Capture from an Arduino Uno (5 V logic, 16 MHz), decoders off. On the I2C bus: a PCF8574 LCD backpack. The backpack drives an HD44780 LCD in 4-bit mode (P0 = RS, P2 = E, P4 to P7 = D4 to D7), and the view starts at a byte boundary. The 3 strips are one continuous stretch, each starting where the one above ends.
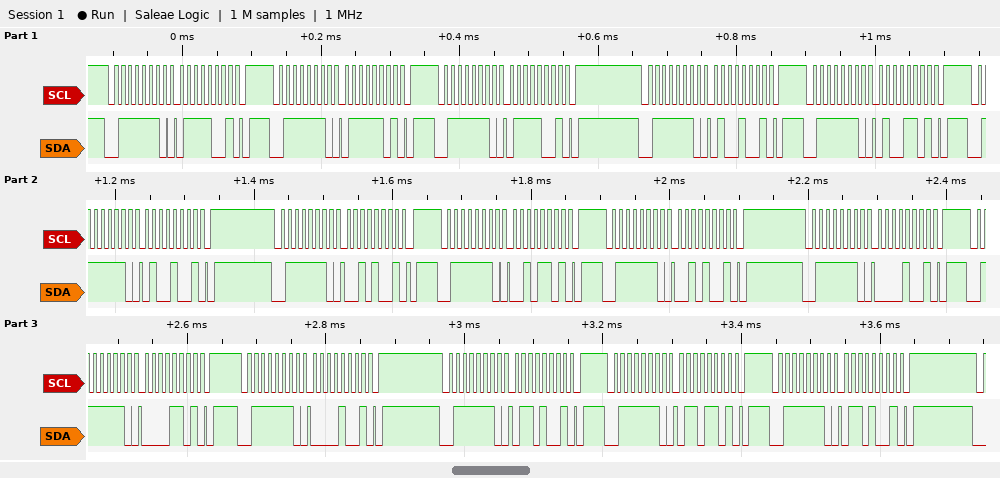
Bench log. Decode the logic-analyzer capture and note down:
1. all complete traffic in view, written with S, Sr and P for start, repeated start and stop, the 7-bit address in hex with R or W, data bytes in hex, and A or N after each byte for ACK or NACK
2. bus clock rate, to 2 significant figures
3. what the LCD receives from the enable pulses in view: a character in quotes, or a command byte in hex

S 3FW A 79 A P S 3FW A 7D A P S 3FW A 79 A P S 3FW A 49 A P S 3FW A 4D A P S 3FW A 49 A P S 3FW A 29 A P S 3FW A 2D A P S 3FW A 29 A P S 3FW A 09 A P S 3FW A 0D A P S 3FW A 09 A P S 3FW A 69 A P S 3FW A 6D A P S 3FW A 69 A P
100 kHz
't' ' '
